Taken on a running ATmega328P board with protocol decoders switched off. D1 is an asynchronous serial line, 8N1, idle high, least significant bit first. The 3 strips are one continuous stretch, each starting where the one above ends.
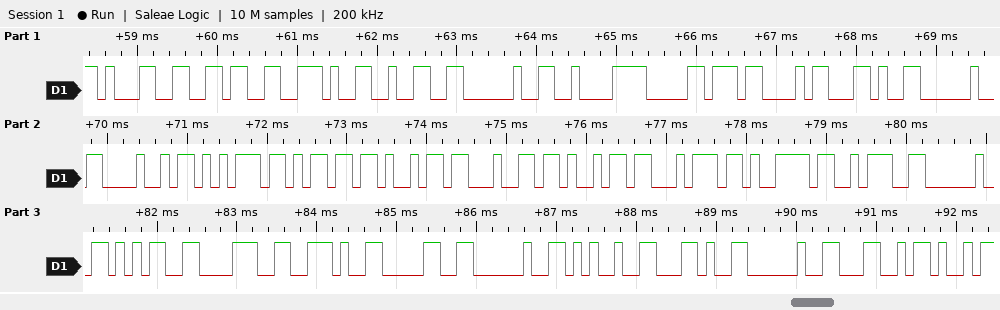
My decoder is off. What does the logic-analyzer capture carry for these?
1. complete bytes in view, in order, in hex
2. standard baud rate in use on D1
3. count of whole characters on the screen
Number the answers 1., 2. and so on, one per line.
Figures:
1. 31 36 2E 32 20 C2 B0 43 2C 20 48 75 6D 69 64 69 74 79 3A 20 35 38 2E 30 20 25 2C 20 4C
2. 9600 baud
3. 29
